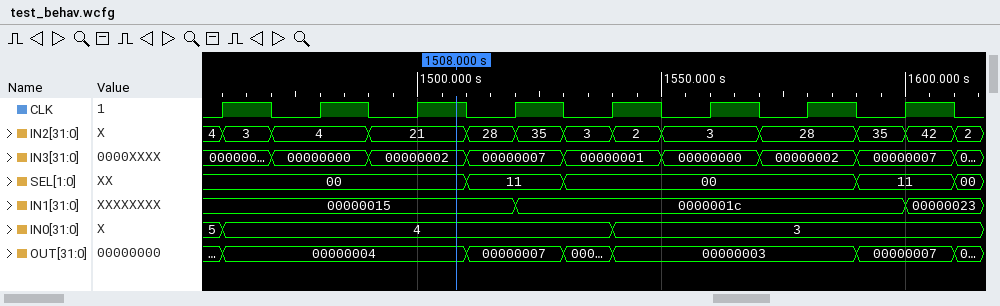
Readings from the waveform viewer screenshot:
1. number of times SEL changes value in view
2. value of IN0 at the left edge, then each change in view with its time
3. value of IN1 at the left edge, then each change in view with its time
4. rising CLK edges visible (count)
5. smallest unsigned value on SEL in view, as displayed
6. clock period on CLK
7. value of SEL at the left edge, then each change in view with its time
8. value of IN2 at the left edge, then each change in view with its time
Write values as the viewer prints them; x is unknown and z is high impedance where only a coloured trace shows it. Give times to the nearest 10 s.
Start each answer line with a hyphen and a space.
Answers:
- 4
- 5, 4 at 1460 s, 3 at 1540 s
- 00000015, 0000001c at 1520 s, 00000023 at 1600 s
- 8
- 00
- 20 s
- 00, 11 at 1510 s, 00 at 1530 s, 11 at 1590 s, 00 at 1610 s
- 4, 3 at 1460 s, 4 at 1470 s, 21 at 1490 s, 28 at 1510 s, 35 at 1520 s, 3 at 1530 s, 2 at 1540 s, 3 at 1550 s, 28 at 1570 s, 35 at 1590 s, 42 at 1600 s, 2 at 1610 s
